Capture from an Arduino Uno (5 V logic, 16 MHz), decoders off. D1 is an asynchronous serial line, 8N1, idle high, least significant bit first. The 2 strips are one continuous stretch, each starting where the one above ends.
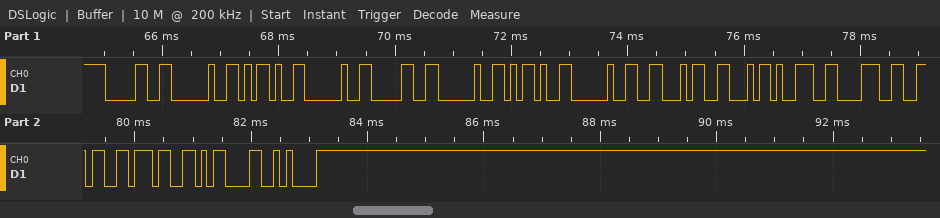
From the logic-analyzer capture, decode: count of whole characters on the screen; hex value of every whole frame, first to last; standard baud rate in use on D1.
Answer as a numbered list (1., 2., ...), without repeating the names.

1. 16
2. 30 20 2D 20 30 20 2D 20 46 46 39 38 36 37 0D 0A
3. 9600 baud
